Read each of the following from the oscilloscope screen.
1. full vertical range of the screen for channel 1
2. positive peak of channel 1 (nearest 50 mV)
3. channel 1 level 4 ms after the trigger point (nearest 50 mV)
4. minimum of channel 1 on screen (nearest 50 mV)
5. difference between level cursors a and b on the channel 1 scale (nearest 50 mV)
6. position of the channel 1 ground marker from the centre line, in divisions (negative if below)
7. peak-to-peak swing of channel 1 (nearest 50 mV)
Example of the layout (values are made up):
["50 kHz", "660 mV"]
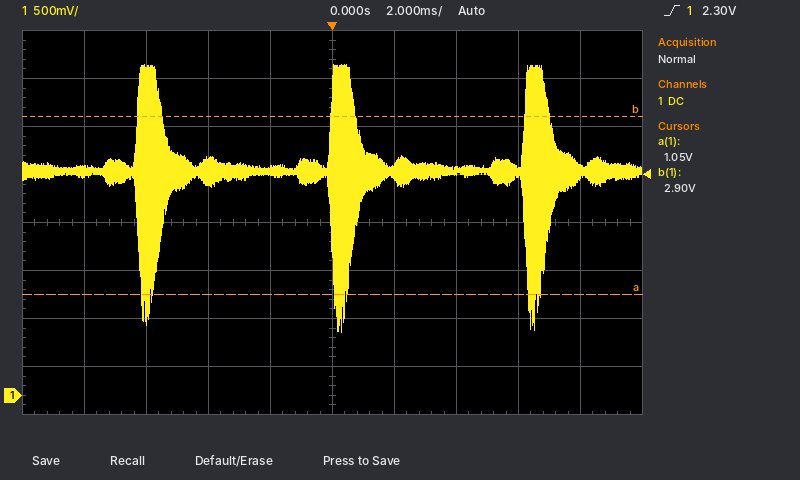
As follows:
["4 V", "3.45 V", "2.35 V", "650 mV", "1.85 V", "-3.6 div", "2.80 V"]
